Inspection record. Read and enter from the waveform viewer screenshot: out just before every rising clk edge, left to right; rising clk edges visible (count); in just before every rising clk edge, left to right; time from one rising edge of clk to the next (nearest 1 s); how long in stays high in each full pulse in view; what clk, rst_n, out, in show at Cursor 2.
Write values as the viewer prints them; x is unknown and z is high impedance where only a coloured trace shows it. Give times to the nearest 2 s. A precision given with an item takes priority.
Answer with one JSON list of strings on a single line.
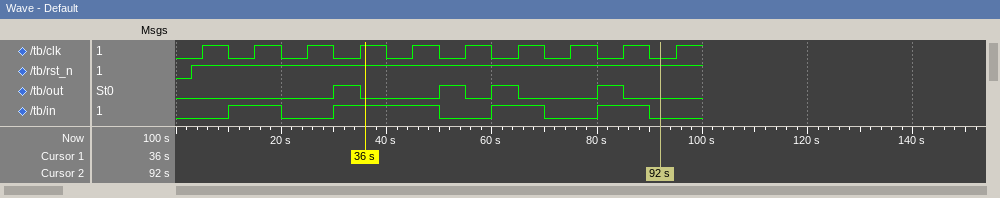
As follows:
["0 0 0 1 0 1 1 0 1 0", "10", "0 1 0 1 1 0 1 0 1 0", "10 s", "10 s, 20 s, 10 s, 10 s", "clk=0, rst_n=1, out=0, in=0"]
